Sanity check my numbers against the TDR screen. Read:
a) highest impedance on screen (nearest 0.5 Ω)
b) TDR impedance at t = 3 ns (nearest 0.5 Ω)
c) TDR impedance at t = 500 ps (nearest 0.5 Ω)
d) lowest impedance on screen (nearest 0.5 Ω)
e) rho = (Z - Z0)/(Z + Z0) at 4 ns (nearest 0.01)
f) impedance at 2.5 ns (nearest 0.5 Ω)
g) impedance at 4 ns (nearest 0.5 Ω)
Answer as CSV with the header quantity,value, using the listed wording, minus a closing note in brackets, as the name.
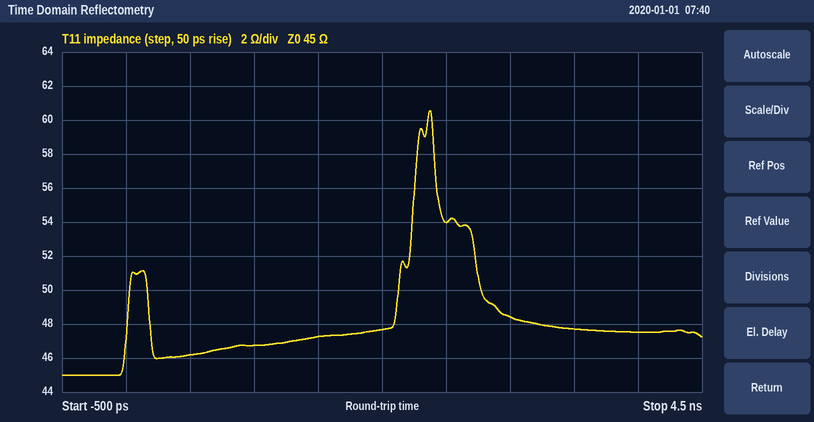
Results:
quantity,value
highest impedance on screen,60.5 Ω
TDR impedance at t = 3 ns,48.5 Ω
TDR impedance at t = 500 ps,46.0 Ω
lowest impedance on screen,45.0 Ω
rho = (Z - Z0)/(Z + Z0) at 4 ns,+0.03
impedance at 2.5 ns,54.0 Ω
impedance at 4 ns,47.5 Ω
